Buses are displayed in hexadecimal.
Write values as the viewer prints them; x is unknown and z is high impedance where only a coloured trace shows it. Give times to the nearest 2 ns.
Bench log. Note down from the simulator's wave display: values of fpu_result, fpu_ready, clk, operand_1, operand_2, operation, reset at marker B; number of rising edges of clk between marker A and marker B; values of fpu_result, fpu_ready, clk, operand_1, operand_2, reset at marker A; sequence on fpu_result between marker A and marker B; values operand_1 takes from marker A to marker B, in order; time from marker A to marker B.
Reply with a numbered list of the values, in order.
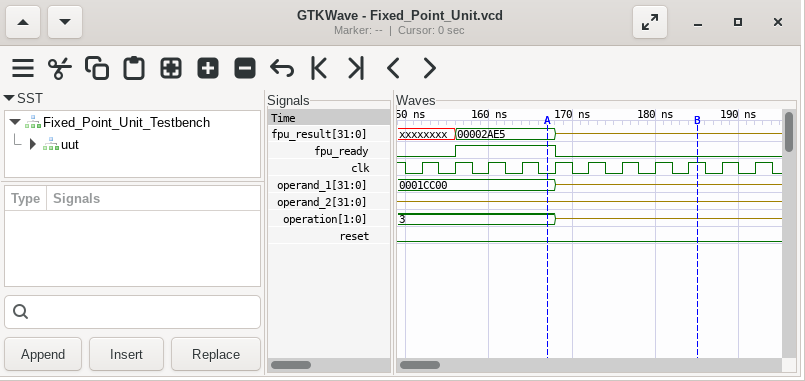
1. fpu_result=z, fpu_ready=0, clk=1, operand_1=z, operand_2=z, operation=z, reset=0
2. 5
3. fpu_result=00002AE5, fpu_ready=1, clk=0, operand_1=0001CC00, operand_2=z, reset=0
4. 00002AE5, z
5. 0001CC00, z
6. 18 ns
